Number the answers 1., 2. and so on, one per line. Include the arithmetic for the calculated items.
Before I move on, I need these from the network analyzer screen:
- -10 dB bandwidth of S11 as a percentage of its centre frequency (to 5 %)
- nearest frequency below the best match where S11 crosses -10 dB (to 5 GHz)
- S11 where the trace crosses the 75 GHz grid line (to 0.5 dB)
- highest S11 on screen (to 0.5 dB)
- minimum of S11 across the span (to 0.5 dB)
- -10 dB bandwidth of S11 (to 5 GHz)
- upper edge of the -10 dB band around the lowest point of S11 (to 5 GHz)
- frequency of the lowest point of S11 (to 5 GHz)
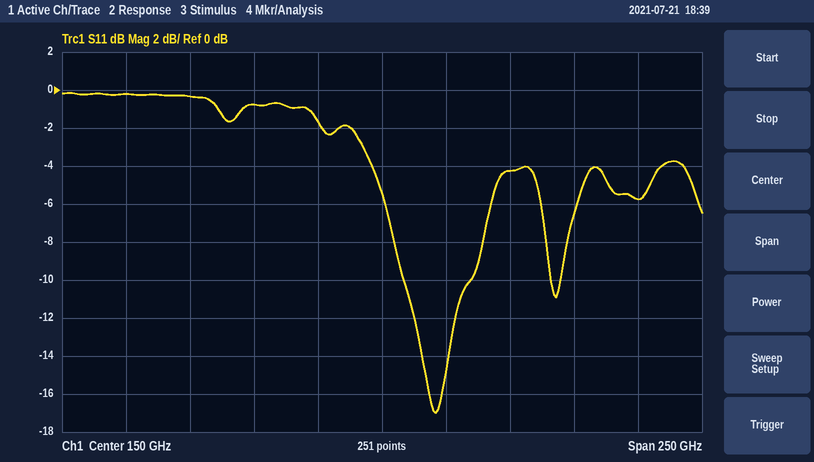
1. 25 GHz / 172.5 GHz ≈ 15 %
2. 160 GHz
3. -0.5 dB
4. 0.0 dB
5. -17.0 dB
6. 185 GHz − 160 GHz = 25 GHz
7. 185 GHz
8. 170 GHz
